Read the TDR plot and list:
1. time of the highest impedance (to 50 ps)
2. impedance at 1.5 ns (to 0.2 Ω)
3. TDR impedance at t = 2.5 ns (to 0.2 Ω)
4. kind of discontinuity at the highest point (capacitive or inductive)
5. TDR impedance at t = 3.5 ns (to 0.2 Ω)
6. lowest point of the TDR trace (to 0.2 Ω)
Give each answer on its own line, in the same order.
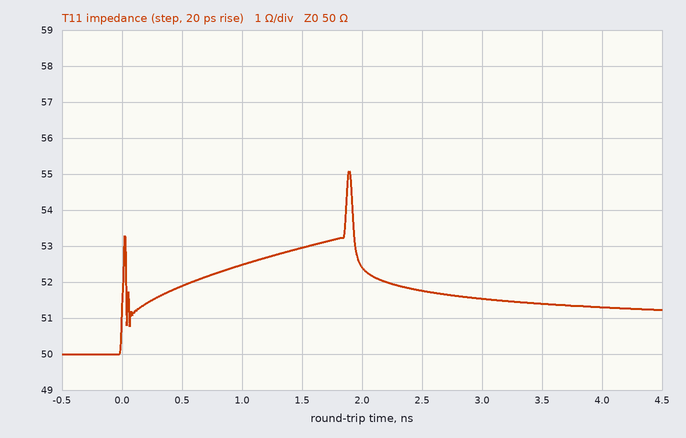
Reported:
1.90 ns
53.0 Ω
51.8 Ω
inductive
51.4 Ω
50.0 Ω
